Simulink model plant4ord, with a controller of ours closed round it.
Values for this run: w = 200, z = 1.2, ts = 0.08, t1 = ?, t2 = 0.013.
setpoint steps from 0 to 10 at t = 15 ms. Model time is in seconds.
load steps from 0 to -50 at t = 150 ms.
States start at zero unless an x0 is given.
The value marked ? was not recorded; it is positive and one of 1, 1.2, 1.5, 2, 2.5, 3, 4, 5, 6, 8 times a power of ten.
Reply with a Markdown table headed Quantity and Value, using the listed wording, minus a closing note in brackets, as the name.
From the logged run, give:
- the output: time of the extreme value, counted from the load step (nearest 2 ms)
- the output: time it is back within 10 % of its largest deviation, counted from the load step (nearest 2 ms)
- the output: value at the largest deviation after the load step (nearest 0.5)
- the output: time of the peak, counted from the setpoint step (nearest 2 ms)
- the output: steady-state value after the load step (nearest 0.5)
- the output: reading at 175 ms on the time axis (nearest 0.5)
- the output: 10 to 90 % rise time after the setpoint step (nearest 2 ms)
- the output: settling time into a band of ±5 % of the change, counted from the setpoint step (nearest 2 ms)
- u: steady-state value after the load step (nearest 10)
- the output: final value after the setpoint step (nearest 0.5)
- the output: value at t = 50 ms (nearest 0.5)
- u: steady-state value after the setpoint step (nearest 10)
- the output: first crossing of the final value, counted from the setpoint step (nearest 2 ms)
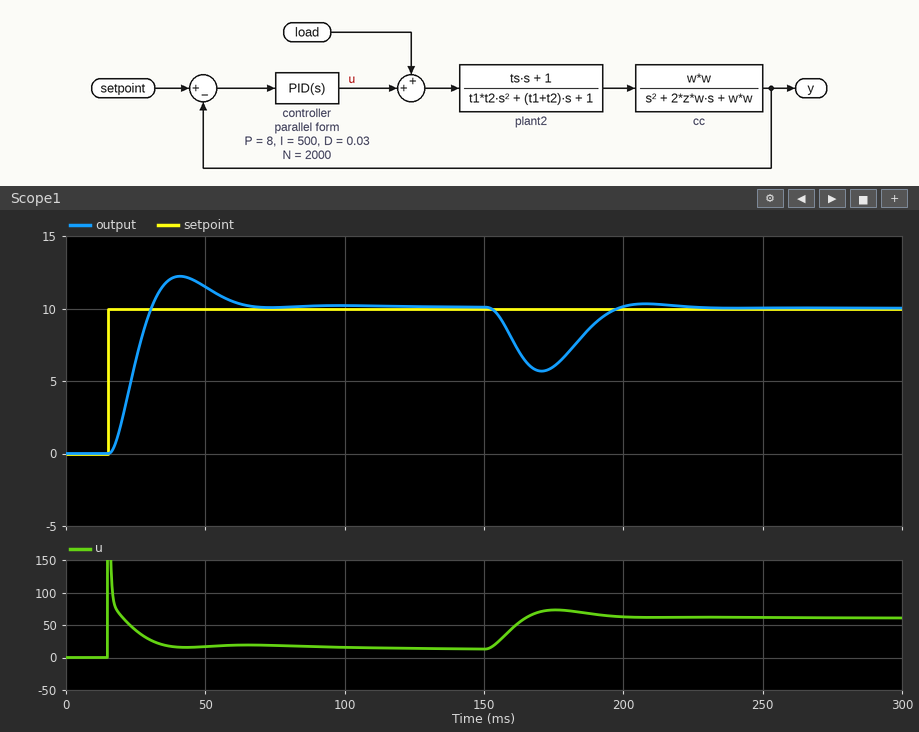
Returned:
| Quantity | Value |
|---|---|
| the output: time of the extreme value, counted from the load step | 20 ms |
| the output: time it is back within 10 % of its largest deviation, counted from the load step | 44 ms |
| the output: value at the largest deviation after the load step | 5.5 |
| the output: time of the peak, counted from the setpoint step | 26 ms |
| the output: steady-state value after the load step | 10.0 |
| the output: reading at 175 ms on the time axis | 6.0 |
| the output: 10 to 90 % rise time after the setpoint step | 10 ms |
| the output: settling time into a band of ±5 % of the change, counted from the setpoint step | 44 ms |
| u: steady-state value after the load step | 60 |
| the output: final value after the setpoint step | 10.0 |
| the output: value at t = 50 ms | 11.5 |
| u: steady-state value after the setpoint step | 10 |
| the output: first crossing of the final value, counted from the setpoint step | 16 ms |
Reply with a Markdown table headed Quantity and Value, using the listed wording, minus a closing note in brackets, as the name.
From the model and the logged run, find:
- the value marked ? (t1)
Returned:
| Quantity | Value |
|---|---|
| the value marked ? | 0.25 |
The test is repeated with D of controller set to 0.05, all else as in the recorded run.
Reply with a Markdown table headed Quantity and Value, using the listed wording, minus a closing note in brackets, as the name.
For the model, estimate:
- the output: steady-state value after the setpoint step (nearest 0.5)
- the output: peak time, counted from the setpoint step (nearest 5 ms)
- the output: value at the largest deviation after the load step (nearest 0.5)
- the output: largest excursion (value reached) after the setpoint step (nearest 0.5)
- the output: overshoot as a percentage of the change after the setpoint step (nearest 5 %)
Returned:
| Quantity | Value |
|---|---|
| the output: steady-state value after the setpoint step | 10.0 |
| the output: peak time, counted from the setpoint step | 30 ms |
| the output: value at the largest deviation after the load step | 6.0 |
| the output: largest excursion (value reached) after the setpoint step | 11.0 |
| the output: overshoot as a percentage of the change after the setpoint step | 10 % |
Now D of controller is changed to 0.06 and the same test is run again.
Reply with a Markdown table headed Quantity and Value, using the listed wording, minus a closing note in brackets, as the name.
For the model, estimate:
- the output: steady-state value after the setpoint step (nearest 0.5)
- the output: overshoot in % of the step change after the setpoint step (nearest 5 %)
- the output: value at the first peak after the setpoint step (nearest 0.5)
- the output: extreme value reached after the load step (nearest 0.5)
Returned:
| Quantity | Value |
|---|---|
| the output: steady-state value after the setpoint step | 10.0 |
| the output: overshoot in % of the step change after the setpoint step | 10 % |
| the output: value at the first peak after the setpoint step | 11.0 |
| the output: extreme value reached after the load step | 6.5 |
